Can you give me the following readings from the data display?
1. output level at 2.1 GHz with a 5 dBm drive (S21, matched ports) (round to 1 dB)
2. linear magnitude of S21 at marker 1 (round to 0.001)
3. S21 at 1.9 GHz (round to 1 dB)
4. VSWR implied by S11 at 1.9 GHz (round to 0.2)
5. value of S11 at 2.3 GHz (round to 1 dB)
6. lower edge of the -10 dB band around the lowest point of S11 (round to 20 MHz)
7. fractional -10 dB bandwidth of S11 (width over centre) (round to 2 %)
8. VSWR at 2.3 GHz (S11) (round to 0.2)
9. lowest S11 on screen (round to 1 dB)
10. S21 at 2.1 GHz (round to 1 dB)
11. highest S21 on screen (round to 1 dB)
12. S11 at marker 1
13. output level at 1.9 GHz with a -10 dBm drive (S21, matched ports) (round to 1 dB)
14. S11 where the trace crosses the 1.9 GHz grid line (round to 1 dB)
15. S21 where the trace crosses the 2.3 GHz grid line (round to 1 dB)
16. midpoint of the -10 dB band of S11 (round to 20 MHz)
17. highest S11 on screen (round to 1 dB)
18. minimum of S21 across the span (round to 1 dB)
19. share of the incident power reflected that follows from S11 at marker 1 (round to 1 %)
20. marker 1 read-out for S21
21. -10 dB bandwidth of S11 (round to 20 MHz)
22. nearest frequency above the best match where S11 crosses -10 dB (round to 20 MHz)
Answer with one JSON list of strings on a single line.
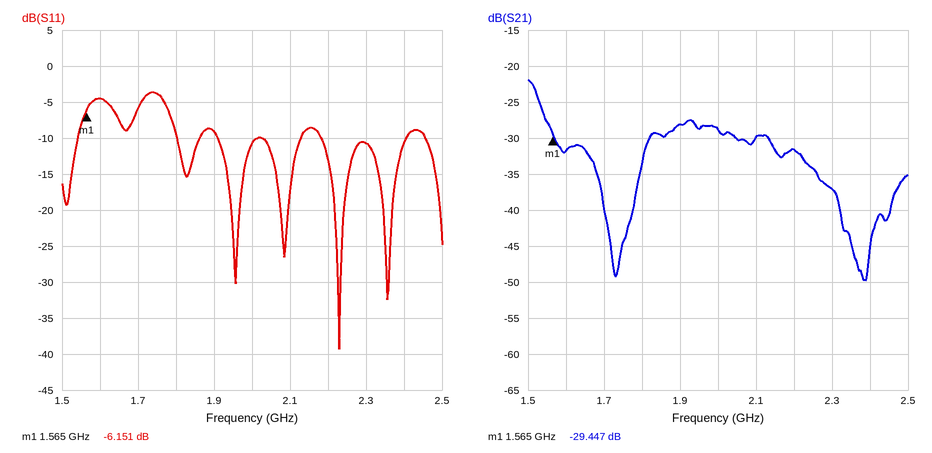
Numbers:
["-25 dBm", "0.034", "-28 dB", "2.0", "-11 dB", "2.18 GHz", "10 %", "1.8", "-39 dB", "-30 dB", "-22 dB", "-6.151 dB", "-38 dBm", "-9 dB", "-37 dB", "2.30 GHz", "-4 dB", "-50 dB", "24 %", "-29.447 dB", "220 MHz", "2.40 GHz"]
